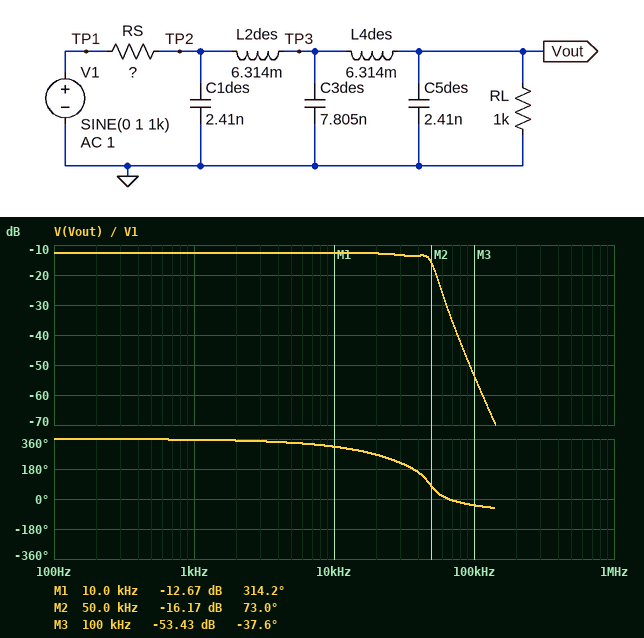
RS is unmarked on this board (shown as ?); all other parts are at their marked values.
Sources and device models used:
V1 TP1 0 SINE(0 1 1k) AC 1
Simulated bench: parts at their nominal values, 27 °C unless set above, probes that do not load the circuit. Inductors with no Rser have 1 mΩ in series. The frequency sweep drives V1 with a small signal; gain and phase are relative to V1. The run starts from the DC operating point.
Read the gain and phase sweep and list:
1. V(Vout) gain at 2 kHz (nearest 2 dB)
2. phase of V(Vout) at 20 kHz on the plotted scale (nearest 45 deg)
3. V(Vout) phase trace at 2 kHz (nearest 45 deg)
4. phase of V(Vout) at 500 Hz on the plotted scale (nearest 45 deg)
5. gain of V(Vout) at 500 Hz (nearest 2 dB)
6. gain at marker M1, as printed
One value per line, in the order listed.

-12 dB
270 deg
360 deg
360 deg
-12 dB
-12.67 dB
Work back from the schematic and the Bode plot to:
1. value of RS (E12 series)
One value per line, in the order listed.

3.3 kΩ
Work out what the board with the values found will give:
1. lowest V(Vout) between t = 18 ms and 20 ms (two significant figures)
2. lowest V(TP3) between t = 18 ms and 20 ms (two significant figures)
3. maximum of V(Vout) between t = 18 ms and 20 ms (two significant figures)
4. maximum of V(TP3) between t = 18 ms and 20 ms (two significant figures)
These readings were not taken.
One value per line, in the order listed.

-230 mV
-230 mV
230 mV
230 mV
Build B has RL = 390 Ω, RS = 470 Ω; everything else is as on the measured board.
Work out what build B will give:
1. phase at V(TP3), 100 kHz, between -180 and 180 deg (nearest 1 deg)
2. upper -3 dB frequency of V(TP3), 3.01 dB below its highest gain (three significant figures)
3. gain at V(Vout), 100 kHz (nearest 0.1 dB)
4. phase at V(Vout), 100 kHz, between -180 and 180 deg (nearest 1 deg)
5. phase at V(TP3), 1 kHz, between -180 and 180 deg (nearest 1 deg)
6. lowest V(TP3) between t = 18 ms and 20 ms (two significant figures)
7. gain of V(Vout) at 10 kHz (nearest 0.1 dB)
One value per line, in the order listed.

150 deg
37.5 kHz
-47.2 dB
34 deg
0 deg
-450 mV
-8.5 dB
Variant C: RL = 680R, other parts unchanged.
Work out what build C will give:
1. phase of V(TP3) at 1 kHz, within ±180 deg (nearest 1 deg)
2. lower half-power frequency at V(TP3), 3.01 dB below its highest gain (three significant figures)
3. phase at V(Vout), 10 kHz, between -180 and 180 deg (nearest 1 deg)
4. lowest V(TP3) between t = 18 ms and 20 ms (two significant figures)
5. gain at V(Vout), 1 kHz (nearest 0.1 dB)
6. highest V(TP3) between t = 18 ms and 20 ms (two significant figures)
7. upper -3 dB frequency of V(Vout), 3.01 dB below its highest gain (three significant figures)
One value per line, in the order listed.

0 deg
18.7 kHz
-40 deg
-170 mV
-15.3 dB
170 mV
45.8 kHz
